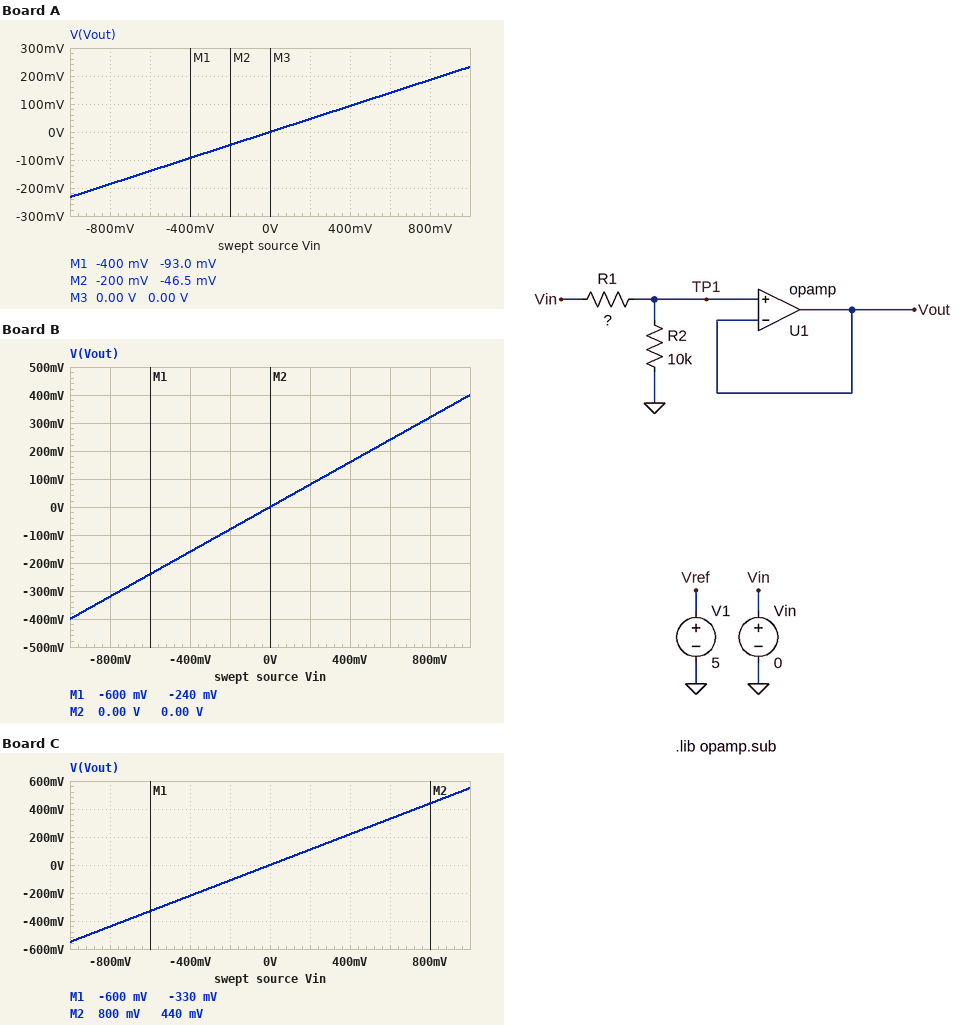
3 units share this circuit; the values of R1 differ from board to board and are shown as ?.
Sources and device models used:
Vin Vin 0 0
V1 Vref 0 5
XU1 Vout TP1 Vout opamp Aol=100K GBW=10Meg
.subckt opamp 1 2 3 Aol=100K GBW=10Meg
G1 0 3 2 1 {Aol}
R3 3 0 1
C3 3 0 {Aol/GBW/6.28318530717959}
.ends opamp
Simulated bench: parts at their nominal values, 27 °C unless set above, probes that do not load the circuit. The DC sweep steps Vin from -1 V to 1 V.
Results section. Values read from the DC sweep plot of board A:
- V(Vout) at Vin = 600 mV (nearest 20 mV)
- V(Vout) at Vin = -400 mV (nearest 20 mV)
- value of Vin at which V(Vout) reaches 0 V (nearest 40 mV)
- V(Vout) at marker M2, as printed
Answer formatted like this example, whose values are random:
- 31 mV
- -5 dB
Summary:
- 140 mV
- -100 mV
- 0 V
- -46.5 mV
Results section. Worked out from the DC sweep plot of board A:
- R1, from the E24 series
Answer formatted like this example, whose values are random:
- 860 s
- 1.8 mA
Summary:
- 33 kΩ
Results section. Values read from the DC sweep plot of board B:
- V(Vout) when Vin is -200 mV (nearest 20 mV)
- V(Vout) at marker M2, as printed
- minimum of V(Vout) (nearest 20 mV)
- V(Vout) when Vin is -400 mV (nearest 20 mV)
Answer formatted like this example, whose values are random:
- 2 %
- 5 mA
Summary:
- -80 mV
- 0.00 V
- -400 mV
- -160 mV
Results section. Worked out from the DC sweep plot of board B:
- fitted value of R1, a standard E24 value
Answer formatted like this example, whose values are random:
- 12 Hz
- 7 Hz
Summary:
- 15 kΩ
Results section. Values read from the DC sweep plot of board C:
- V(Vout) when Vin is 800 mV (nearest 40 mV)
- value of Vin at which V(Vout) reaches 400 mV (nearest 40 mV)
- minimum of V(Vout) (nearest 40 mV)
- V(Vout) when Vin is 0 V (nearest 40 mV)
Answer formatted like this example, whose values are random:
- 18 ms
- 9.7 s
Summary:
- 440 mV
- 720 mV
- -560 mV
- 0 V
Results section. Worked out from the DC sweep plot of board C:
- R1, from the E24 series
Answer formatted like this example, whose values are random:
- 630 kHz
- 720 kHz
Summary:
- 8.2 kΩ
